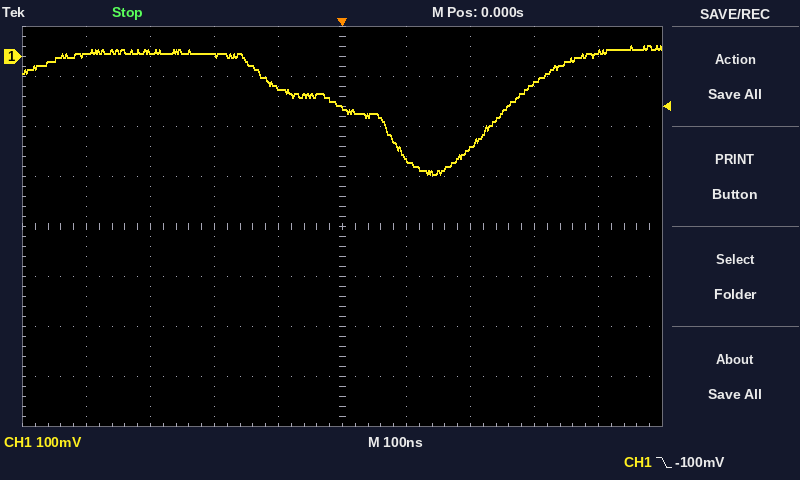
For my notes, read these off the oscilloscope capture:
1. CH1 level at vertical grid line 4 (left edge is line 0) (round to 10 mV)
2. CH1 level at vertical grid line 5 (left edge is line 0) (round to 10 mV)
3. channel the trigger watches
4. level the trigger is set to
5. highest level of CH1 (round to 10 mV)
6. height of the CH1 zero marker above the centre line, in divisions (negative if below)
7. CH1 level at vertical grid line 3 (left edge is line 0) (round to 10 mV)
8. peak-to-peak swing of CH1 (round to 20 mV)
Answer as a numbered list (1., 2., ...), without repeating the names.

1. -60 mV
2. -100 mV
3. CH1
4. -100 mV
5. 20 mV
6. +3.4 div
7. 0 mV
8. 260 mV
